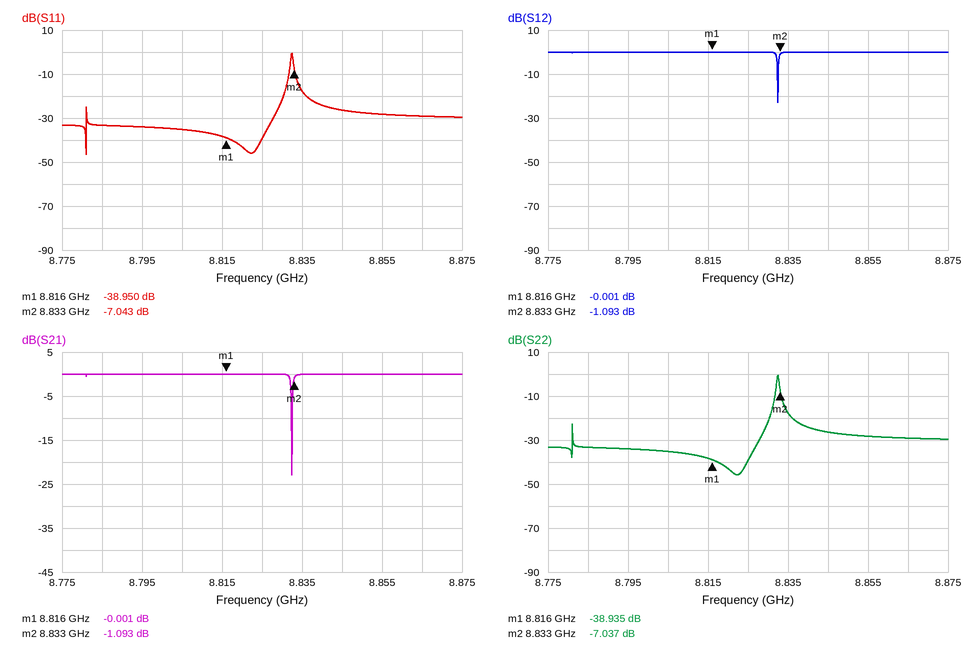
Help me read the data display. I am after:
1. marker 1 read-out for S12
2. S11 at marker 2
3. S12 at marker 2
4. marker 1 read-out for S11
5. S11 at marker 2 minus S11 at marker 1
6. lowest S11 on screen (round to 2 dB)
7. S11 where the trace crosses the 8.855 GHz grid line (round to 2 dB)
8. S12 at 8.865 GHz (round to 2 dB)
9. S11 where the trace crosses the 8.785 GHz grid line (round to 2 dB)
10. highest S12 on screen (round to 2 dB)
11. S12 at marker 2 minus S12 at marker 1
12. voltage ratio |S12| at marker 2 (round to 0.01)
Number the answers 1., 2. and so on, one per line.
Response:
1. -0.001 dB
2. -7.043 dB
3. -1.093 dB
4. -38.950 dB
5. 31.907 dB
6. -46 dB
7. -28 dB
8. 0 dB
9. -34 dB
10. 0 dB
11. -1.092 dB
12. 0.88
